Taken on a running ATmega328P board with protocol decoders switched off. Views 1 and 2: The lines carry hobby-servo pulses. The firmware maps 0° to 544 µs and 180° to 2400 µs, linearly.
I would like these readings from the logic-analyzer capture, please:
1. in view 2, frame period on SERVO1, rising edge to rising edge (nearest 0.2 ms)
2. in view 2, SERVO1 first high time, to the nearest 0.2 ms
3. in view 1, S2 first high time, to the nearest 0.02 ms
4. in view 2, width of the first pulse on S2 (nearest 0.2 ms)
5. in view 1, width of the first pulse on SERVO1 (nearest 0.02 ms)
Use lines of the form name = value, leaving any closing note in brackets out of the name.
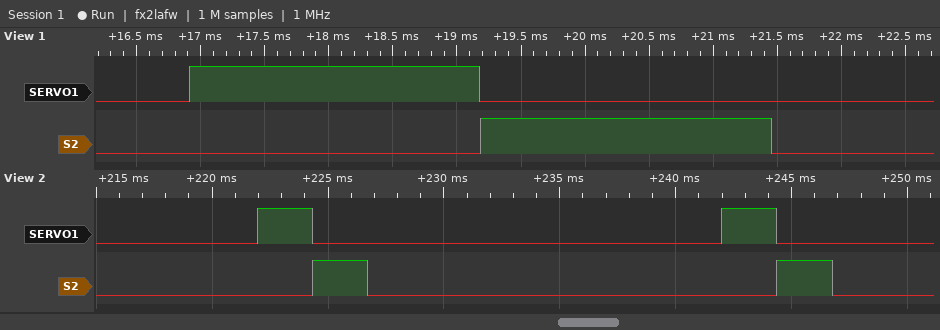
in view 2, frame period on SERVO1, rising edge to rising edge = 20.0 ms
in view 2, SERVO1 first high time, to the nearest 0.2 ms = 2.4 ms
in view 1, S2 first high time, to the nearest 0.02 ms = 2.26 ms
in view 2, width of the first pulse on S2 = 2.4 ms
in view 1, width of the first pulse on SERVO1 = 2.26 ms
